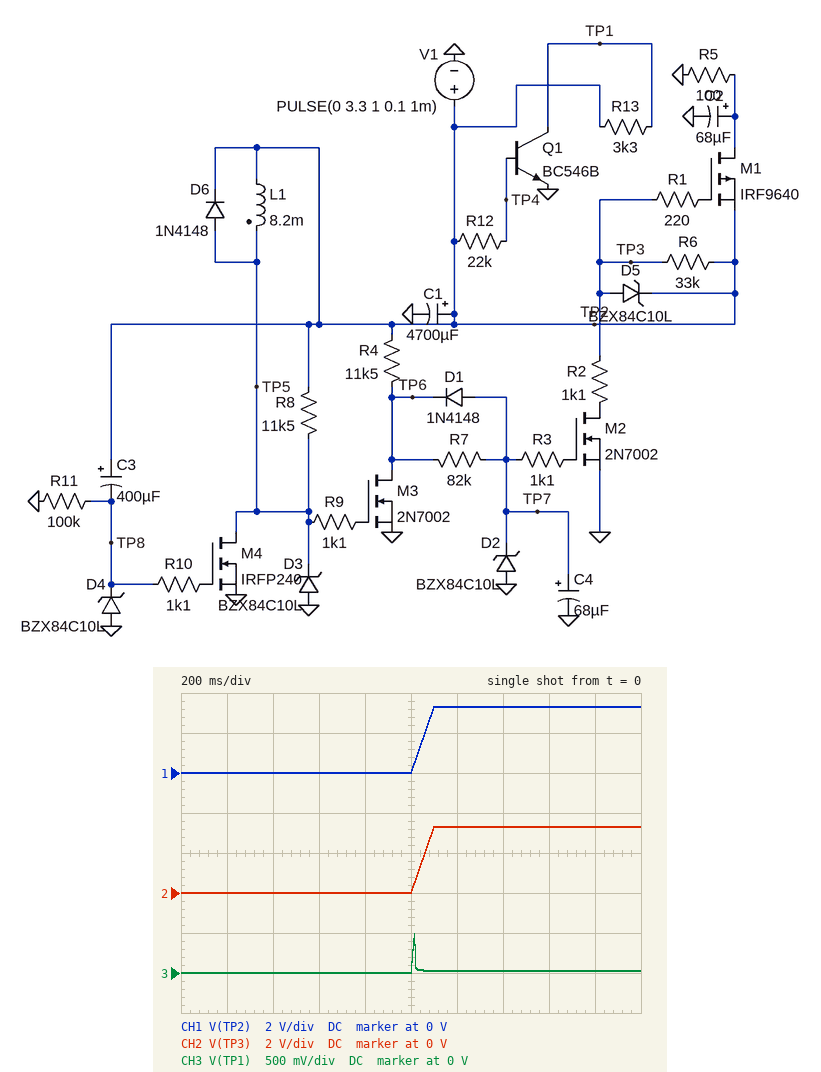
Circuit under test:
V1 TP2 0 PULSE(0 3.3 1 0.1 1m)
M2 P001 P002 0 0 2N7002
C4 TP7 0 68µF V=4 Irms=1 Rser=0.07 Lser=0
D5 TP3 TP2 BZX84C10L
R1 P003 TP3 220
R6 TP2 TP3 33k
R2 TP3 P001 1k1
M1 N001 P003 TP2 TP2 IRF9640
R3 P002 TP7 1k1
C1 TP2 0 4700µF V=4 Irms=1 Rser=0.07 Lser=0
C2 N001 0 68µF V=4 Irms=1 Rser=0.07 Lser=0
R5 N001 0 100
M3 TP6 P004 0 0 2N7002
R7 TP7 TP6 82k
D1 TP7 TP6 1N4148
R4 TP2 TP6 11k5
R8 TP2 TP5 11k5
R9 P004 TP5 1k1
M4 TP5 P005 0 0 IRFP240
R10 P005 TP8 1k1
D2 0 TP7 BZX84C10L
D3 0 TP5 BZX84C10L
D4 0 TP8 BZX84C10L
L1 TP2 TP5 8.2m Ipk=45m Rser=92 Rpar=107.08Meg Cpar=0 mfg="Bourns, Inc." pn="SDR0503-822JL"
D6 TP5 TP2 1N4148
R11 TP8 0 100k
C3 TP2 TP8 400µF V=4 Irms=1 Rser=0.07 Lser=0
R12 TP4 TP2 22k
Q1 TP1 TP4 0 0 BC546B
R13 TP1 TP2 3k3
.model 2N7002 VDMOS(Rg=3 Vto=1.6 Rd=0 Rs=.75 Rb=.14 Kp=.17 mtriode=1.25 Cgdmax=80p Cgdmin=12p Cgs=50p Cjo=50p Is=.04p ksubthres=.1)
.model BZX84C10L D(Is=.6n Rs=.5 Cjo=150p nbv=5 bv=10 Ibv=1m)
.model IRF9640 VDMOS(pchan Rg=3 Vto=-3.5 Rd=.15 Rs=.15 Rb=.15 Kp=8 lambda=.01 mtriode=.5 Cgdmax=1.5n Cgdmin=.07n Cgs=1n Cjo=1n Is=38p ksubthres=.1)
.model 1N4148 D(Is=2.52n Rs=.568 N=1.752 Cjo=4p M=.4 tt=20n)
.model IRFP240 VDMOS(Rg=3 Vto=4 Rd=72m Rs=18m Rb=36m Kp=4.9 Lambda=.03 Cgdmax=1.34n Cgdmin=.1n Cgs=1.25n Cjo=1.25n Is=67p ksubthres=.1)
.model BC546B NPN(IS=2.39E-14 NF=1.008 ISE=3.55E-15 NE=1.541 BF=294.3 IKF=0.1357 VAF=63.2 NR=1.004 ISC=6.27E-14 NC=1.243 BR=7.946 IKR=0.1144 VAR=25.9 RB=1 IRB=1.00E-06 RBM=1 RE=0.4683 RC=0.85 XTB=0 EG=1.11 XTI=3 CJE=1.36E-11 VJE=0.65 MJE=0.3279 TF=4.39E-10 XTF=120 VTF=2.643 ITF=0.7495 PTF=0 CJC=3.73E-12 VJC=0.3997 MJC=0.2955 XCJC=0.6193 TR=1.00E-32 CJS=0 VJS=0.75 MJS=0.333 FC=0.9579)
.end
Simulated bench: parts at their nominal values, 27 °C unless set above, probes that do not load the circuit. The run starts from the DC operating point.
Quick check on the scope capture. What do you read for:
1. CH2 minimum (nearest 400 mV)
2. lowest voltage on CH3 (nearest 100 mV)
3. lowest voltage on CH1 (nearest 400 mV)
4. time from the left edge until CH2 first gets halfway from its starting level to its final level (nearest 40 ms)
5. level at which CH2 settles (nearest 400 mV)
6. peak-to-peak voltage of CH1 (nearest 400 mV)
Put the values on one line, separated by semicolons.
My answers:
0 V; 0 V; 0 V; 1.04 s; 3.2 V; 3.2 V
